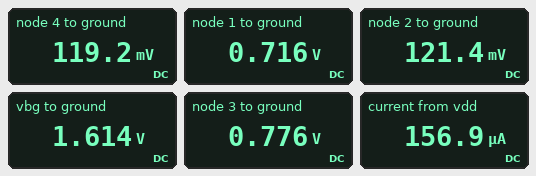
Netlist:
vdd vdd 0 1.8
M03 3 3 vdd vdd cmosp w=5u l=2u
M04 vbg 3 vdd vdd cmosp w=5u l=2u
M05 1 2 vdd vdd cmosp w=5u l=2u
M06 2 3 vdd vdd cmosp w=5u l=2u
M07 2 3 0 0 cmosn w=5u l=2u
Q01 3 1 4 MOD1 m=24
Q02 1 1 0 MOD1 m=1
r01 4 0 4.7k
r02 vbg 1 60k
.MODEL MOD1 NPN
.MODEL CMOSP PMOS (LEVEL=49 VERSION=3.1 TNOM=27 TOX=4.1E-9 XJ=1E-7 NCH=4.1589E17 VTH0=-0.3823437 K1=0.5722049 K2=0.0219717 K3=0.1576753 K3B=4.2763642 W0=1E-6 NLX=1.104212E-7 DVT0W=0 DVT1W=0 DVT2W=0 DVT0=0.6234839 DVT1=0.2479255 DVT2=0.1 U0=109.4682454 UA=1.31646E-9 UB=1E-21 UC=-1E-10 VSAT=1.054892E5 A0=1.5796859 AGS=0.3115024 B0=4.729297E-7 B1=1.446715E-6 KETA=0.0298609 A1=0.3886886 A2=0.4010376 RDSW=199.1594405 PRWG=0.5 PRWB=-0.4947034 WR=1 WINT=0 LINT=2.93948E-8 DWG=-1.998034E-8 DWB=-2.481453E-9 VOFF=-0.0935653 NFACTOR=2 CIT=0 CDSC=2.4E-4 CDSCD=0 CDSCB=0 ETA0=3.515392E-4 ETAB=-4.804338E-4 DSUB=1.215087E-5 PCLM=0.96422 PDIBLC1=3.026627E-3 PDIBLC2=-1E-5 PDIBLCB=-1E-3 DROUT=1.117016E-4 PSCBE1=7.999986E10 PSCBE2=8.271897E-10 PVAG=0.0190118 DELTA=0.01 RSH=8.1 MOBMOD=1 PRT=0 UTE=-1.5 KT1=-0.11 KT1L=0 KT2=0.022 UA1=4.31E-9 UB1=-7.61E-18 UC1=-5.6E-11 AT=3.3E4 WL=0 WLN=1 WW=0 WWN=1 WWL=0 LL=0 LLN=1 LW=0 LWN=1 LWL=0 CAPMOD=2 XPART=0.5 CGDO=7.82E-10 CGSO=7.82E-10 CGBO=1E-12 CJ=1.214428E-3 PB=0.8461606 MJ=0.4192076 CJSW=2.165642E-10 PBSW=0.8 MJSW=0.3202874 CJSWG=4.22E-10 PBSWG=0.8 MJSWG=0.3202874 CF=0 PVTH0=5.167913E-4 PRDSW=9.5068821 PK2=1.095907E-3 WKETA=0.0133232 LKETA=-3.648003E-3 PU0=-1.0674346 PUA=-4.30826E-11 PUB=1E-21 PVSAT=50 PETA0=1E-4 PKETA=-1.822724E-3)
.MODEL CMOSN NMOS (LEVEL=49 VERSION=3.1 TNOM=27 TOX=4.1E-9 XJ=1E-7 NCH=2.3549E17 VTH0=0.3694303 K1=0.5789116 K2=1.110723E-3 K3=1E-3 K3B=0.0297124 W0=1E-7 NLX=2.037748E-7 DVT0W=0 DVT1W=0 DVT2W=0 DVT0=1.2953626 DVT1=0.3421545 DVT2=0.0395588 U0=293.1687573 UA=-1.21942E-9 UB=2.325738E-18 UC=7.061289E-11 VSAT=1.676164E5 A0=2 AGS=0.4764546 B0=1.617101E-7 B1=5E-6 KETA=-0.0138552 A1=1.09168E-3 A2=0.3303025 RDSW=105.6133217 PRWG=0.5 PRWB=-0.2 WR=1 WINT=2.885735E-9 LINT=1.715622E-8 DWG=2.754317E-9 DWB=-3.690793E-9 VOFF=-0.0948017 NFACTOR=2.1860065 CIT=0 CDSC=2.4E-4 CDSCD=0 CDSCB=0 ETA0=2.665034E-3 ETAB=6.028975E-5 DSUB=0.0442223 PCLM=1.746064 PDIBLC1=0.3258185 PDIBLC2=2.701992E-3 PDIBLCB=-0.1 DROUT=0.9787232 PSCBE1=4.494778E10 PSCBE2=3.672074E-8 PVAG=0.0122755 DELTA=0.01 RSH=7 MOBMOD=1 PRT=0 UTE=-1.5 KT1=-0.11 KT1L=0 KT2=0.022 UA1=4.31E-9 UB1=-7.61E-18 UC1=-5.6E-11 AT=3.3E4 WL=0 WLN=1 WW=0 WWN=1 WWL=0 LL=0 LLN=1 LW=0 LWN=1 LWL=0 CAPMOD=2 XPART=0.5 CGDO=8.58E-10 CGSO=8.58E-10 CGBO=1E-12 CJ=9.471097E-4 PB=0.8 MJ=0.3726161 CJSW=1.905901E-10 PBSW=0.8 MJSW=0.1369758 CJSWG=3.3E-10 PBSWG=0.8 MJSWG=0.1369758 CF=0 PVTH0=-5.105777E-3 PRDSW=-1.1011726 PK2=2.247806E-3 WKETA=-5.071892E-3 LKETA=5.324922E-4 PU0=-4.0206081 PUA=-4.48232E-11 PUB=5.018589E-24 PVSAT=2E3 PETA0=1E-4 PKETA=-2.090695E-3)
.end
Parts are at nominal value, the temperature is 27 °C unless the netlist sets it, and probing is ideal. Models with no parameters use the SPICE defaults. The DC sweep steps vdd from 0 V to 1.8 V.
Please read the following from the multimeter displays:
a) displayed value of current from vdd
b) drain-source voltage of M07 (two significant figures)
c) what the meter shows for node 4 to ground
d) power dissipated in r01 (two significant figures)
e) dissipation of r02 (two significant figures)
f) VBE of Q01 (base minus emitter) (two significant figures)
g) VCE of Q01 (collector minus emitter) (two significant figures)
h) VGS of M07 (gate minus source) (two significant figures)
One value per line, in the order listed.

156.9 µA
120 mV
119.2 mV
3.0 µW
13 µW
600 mV
660 mV
780 mV
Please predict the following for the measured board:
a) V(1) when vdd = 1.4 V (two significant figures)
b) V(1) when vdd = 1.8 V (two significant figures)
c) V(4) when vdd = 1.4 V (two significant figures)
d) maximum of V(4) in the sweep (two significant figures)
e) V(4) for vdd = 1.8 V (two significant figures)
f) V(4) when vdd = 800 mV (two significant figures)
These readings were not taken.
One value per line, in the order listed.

650 mV
720 mV
71 mV
120 mV
120 mV
36 mV
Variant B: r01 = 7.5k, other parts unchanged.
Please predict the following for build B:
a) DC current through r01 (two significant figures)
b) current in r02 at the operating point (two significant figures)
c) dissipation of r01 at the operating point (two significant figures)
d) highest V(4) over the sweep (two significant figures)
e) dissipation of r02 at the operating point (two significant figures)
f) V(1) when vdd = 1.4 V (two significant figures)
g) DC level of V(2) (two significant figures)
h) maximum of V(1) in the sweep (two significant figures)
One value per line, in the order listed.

17 µA
14 µA
2.3 µW
130 mV
12 µW
660 mV
54 mV
720 mV
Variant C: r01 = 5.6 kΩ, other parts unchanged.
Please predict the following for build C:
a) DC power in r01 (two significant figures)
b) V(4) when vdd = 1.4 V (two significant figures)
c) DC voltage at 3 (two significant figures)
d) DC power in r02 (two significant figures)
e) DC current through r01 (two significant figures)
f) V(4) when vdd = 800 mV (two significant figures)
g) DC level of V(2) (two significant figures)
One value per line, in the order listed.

2.7 µW
73 mV
820 mV
13 µW
22 µA
40 mV
86 mV
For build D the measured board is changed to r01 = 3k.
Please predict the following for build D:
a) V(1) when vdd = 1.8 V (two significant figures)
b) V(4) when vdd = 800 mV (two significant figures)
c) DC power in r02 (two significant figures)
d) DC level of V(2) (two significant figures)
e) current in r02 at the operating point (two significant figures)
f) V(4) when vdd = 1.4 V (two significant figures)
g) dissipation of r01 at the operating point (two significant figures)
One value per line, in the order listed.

690 mV
26 mV
15 µW
790 mV
16 µA
63 mV
2.7 µW
